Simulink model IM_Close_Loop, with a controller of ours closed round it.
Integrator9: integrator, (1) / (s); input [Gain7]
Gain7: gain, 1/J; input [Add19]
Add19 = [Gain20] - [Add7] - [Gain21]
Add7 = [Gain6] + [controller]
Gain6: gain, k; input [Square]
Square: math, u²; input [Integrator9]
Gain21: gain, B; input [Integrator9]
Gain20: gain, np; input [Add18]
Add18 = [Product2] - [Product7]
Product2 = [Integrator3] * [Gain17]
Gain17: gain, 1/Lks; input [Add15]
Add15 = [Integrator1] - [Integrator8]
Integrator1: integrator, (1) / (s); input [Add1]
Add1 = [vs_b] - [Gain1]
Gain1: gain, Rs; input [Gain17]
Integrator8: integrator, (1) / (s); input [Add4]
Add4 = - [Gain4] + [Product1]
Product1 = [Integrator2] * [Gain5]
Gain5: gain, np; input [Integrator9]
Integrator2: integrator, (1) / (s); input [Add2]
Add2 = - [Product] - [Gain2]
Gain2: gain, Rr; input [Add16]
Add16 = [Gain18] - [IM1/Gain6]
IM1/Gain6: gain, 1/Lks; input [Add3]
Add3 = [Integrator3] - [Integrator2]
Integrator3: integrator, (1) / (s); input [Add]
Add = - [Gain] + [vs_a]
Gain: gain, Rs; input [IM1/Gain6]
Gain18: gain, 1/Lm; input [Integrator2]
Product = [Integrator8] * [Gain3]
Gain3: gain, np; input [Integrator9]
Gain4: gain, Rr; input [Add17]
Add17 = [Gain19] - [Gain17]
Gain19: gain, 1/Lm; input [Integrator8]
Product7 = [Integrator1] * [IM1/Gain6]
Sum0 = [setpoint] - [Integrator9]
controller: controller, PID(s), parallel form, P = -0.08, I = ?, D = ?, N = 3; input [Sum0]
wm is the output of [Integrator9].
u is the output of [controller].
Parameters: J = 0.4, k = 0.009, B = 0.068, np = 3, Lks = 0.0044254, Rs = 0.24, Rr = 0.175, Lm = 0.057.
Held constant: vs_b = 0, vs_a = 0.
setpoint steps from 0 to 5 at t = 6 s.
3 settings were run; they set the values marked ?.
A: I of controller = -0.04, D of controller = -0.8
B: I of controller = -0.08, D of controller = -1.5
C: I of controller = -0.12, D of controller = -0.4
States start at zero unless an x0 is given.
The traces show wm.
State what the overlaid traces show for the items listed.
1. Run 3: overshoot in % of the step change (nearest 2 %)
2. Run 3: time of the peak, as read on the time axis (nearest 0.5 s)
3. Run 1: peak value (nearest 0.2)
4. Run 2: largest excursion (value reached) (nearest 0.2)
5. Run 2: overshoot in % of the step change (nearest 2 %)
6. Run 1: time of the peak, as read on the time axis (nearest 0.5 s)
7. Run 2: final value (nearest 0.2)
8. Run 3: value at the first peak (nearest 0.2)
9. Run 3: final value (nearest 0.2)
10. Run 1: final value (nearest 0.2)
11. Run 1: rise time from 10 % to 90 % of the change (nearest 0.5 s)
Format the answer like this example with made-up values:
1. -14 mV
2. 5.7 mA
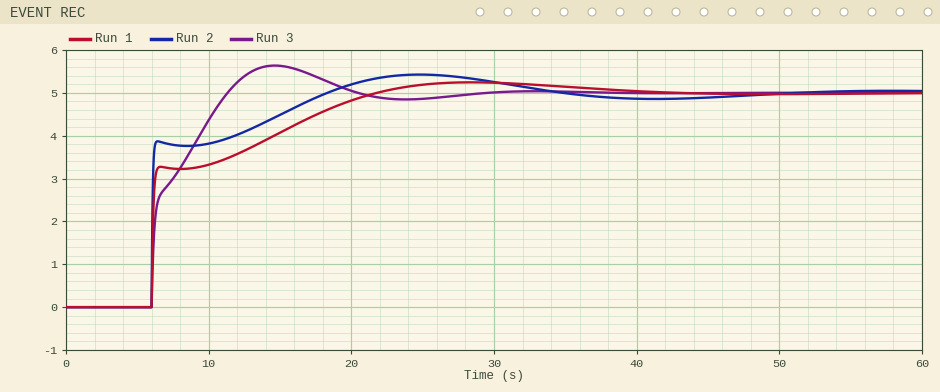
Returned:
1. 12 %
2. 14.5 s
3. 5.2
4. 5.4
5. 8 %
6. 28.5 s
7. 5.0
8. 5.6
9. 5.0
10. 5.0
11. 11.5 s
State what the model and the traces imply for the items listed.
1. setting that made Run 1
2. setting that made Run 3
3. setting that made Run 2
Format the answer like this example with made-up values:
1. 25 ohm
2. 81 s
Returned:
1. A
2. C
3. B
